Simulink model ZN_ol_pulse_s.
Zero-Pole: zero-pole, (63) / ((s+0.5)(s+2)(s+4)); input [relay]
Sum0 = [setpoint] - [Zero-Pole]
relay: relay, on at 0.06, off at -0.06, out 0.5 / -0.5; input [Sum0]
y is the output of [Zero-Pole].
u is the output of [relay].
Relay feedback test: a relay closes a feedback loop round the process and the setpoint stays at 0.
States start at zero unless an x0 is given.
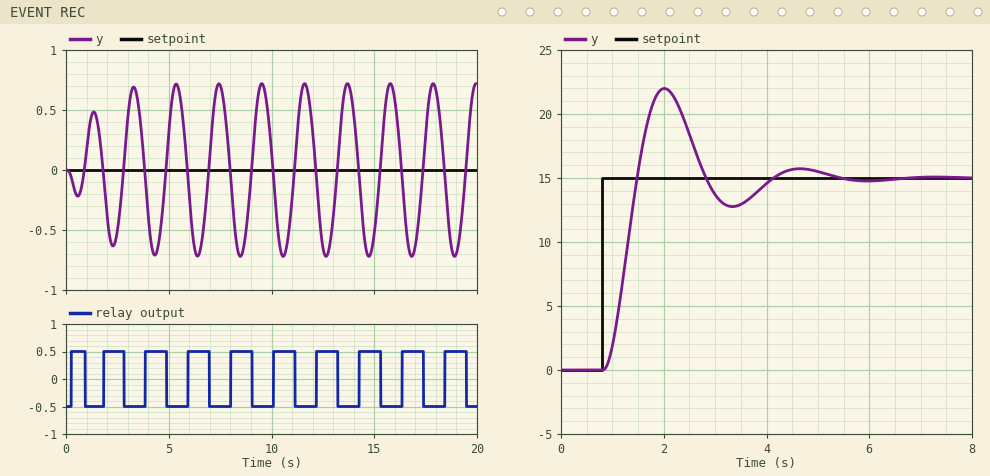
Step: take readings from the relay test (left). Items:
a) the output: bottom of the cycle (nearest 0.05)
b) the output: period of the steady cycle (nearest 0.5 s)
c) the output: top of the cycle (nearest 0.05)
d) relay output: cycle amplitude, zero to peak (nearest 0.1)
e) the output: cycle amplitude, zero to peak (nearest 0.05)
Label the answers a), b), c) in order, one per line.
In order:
a) -0.70
b) 2.0 s
c) 0.70
d) 0.5
e) 0.70
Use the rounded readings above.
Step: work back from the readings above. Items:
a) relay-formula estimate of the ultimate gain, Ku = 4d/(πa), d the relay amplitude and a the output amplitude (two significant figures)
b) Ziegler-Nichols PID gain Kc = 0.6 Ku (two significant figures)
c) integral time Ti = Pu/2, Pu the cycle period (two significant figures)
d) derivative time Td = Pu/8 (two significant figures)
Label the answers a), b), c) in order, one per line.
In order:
a) 0.91
b) 0.55
c) 1.0 s
d) 0.25 s
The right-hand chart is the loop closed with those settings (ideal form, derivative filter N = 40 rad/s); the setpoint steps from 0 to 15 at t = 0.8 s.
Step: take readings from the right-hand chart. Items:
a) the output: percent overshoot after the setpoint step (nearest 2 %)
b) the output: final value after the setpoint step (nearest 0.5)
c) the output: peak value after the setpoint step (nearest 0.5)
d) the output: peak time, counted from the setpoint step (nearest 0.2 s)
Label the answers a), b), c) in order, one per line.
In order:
a) 46 %
b) 15.0
c) 22.0
d) 1.2 s
